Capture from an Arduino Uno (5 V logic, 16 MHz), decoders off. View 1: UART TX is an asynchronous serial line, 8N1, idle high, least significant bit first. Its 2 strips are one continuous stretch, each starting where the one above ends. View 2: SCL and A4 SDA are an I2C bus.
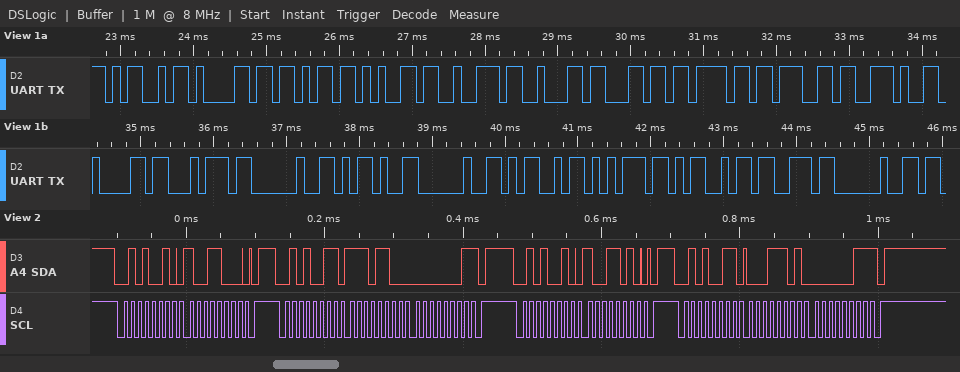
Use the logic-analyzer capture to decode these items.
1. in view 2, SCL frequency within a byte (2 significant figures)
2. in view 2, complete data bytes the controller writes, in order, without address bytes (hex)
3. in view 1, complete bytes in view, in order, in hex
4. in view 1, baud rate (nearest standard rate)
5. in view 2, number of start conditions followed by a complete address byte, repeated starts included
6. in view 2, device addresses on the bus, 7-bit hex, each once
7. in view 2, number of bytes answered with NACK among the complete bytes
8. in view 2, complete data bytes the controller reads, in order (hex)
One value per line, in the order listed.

100 kHz
98 9A
4D 61 6B 65 72 62 6C 6F 67 2E 61 74 20 2D 20 4D 75 4D 73 20
9600 baud
4
0x29
2
EC 01 1D 03
